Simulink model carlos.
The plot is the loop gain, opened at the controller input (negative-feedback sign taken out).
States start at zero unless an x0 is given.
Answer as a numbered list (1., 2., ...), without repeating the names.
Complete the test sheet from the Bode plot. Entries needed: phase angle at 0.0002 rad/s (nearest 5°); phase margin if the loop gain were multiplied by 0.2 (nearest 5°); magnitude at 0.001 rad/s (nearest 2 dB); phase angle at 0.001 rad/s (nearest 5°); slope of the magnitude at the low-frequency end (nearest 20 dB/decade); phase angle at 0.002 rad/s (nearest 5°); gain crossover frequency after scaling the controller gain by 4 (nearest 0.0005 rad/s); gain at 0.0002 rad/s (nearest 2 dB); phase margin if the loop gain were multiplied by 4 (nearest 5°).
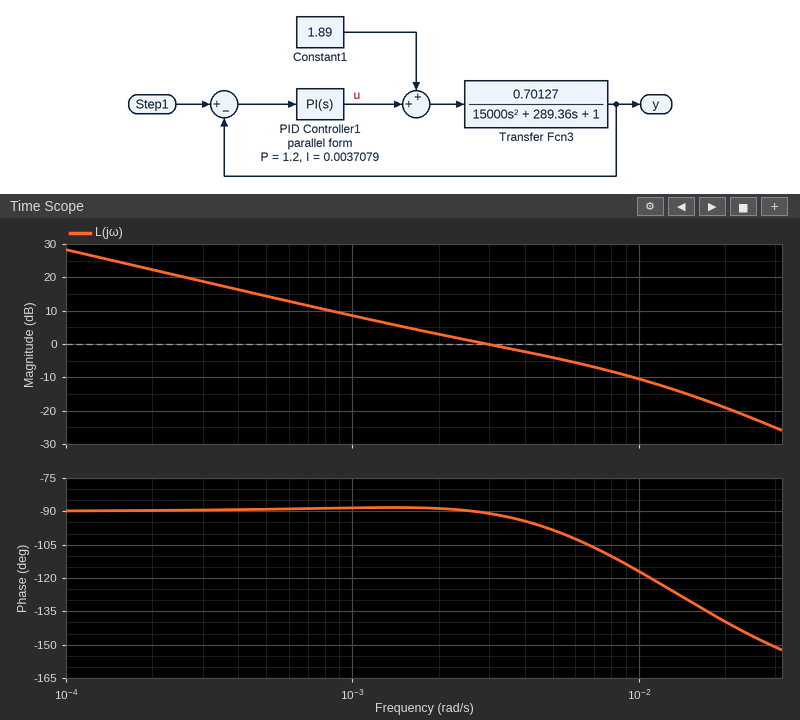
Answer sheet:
1. -90°
2. 90°
3. 8 dB
4. -90°
5. -20 dB/decade
6. -90°
7. 0.0115 rad/s
8. 22 dB
9. 60°
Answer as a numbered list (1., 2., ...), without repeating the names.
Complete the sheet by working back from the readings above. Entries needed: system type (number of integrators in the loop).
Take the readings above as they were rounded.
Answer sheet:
1. 1
